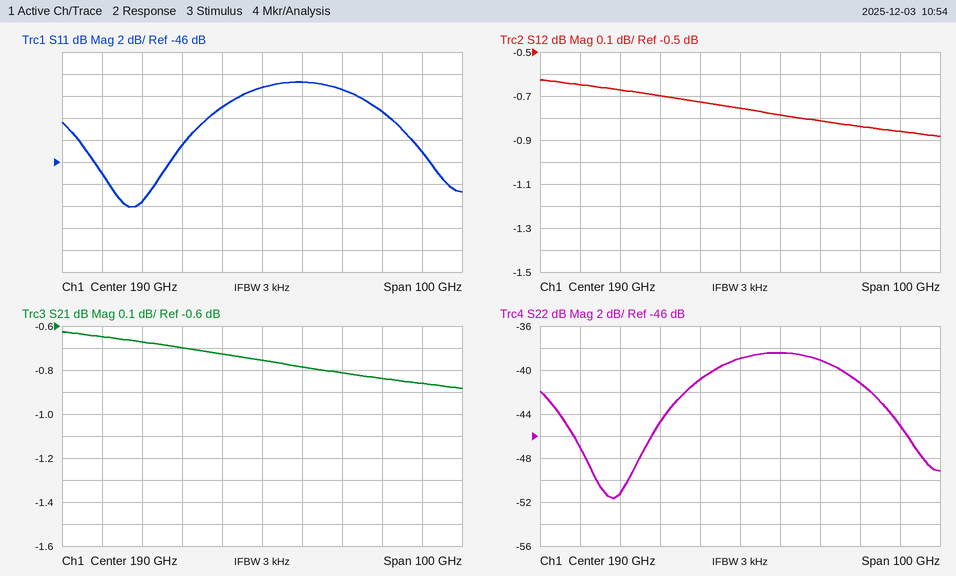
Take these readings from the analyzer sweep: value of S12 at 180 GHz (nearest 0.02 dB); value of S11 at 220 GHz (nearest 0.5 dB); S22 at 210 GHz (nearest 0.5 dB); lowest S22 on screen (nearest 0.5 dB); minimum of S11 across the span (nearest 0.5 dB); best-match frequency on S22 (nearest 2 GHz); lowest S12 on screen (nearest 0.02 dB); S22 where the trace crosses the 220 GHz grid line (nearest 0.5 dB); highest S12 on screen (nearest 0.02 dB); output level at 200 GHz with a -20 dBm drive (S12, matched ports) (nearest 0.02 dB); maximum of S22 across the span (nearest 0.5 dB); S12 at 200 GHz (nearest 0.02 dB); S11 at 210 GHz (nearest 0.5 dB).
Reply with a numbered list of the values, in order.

1. -0.72 dB
2. -41.5 dB
3. -39.0 dB
4. -51.5 dB
5. -50.0 dB
6. 158 GHz
7. -0.88 dB
8. -41.0 dB
9. -0.62 dB
10. -20.78 dBm
11. -38.5 dB
12. -0.78 dB
13. -39.5 dB
